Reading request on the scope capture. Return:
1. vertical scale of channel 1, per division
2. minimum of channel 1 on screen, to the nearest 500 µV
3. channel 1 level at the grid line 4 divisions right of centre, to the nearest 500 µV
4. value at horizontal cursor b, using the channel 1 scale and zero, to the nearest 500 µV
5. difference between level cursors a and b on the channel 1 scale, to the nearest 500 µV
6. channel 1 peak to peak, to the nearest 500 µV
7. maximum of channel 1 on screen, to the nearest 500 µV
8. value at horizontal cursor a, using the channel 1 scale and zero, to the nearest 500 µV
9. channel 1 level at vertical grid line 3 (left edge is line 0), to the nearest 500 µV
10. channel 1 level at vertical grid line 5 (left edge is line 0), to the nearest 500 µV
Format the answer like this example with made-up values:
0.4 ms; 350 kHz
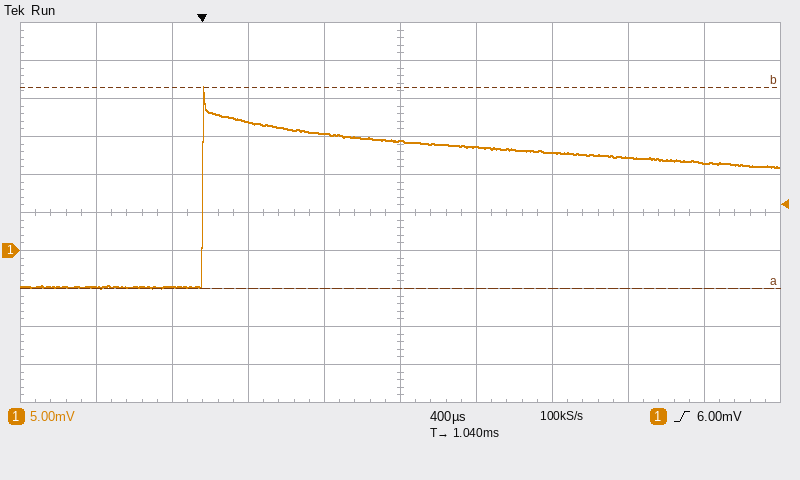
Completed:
5 mV; -5.0 mV; 11.5 mV; 21.5 mV; 26.5 mV; 26.5 mV; 21.5 mV; -5.0 mV; 17.0 mV; 14.5 mV
